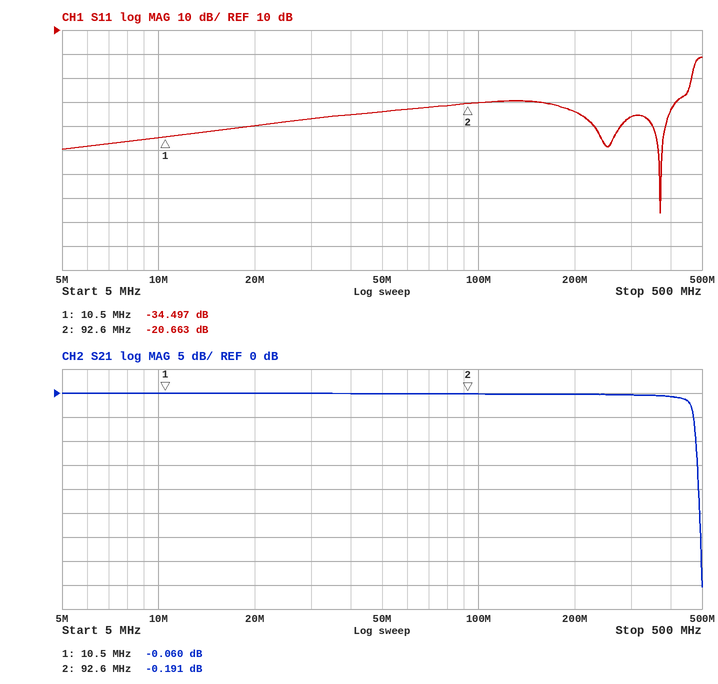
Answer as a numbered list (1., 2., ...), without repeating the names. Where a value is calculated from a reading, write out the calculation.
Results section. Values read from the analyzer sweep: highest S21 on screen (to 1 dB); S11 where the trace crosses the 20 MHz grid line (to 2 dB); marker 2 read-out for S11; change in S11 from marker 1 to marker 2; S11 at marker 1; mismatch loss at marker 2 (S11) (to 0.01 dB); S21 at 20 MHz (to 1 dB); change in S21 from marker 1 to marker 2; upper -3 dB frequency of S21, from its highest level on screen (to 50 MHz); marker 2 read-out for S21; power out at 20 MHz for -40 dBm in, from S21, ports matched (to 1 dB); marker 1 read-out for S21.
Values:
1. 0 dB
2. -30 dB
3. -20.663 dB
4. -20.663 − (-34.497) = 13.834 dB
5. -34.497 dB
6. −10 log10(1 − 10^(-20.663/10)) ≈ 0.04 dB
7. 0 dB
8. -0.191 − (-0.06) = -0.131 dB
9. 450 MHz
10. -0.191 dB
11. -40 dBm + (0 dB) = -40 dBm
12. -0.060 dB
